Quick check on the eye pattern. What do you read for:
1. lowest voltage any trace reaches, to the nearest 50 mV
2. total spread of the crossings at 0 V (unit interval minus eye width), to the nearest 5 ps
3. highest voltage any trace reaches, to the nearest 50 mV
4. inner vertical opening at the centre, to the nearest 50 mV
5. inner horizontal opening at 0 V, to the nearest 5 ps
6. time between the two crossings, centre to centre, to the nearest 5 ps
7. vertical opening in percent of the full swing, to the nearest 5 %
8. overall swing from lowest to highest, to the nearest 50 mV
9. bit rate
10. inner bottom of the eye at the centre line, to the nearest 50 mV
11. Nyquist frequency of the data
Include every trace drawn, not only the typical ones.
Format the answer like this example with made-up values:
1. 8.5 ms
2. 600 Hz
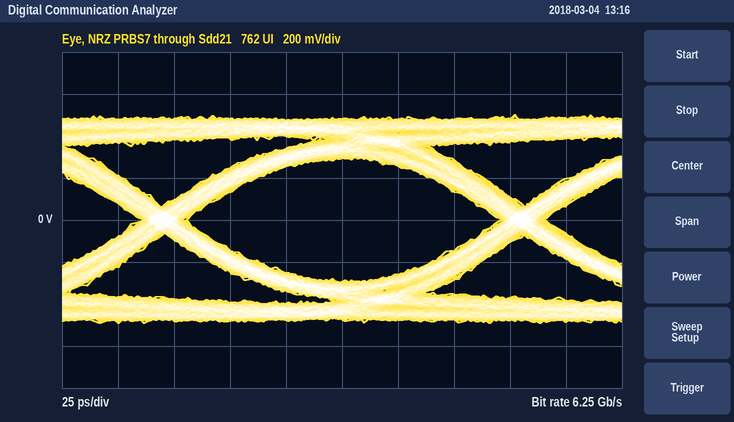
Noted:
1. -500 mV
2. 20 ps
3. 500 mV
4. 600 mV
5. 140 ps
6. 160 ps
7. 60 %
8. 1.00 V
9. 6.25 Gb/s
10. -300 mV
11. 3.125 GHz
